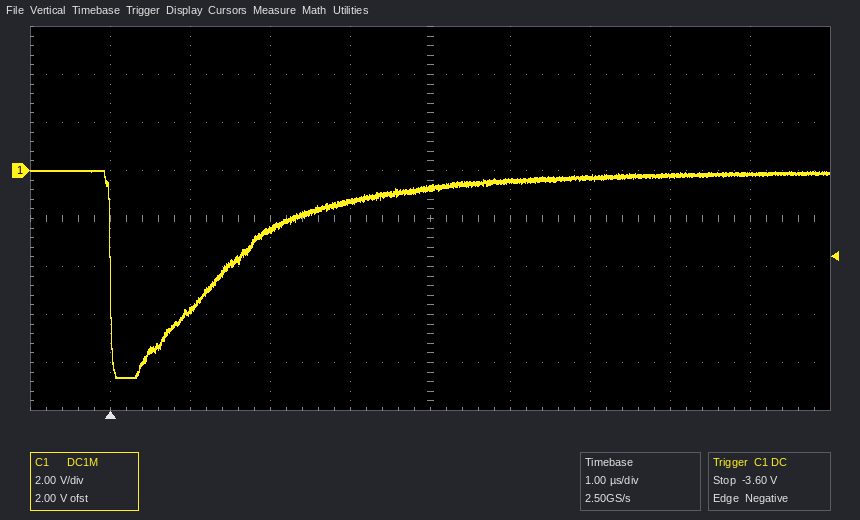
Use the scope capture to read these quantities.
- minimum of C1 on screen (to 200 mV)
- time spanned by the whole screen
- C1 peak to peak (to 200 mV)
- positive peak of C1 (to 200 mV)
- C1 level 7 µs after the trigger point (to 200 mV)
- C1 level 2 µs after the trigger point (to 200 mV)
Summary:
-8.6 V
10 µs
8.6 V
0.0 V
-200 mV
-2.4 V
